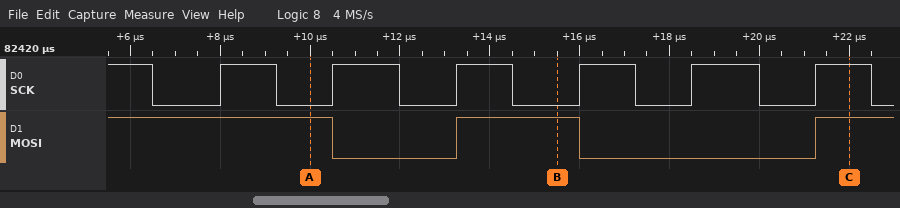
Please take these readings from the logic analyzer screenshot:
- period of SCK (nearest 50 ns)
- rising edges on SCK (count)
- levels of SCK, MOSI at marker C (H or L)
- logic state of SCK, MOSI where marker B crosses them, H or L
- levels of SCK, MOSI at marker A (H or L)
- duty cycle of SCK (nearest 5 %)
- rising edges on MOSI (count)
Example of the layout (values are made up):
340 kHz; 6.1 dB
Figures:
2650 ns; 6; SCK=H, MOSI=H; SCK=L, MOSI=H; SCK=L, MOSI=H; 50 %; 2
